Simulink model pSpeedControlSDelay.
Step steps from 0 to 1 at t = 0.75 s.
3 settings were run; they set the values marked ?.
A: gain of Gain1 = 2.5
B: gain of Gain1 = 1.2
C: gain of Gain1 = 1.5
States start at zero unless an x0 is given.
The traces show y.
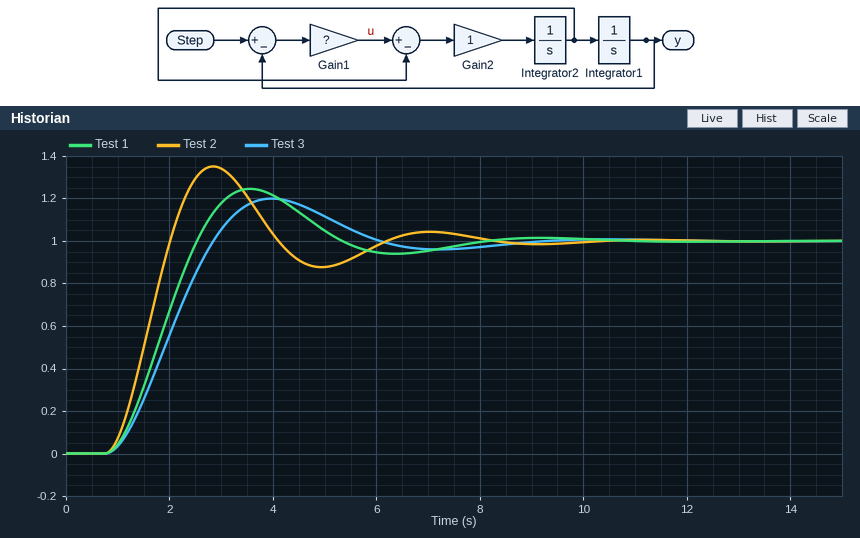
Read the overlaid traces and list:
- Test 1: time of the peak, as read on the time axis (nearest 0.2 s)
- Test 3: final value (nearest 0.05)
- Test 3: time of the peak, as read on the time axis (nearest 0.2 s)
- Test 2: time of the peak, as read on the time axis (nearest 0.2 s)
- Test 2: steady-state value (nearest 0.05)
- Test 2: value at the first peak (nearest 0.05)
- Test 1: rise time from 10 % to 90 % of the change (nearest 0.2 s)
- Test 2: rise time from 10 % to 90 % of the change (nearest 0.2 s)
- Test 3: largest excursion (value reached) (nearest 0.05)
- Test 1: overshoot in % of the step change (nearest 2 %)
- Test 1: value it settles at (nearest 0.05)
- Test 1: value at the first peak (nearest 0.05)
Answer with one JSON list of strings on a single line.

["3.6 s", "1.00", "4.0 s", "2.8 s", "1.00", "1.35", "1.2 s", "0.8 s", "1.20", "24 %", "1.00", "1.25"]
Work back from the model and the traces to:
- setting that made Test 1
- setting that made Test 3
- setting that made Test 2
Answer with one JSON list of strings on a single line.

["C", "B", "A"]
